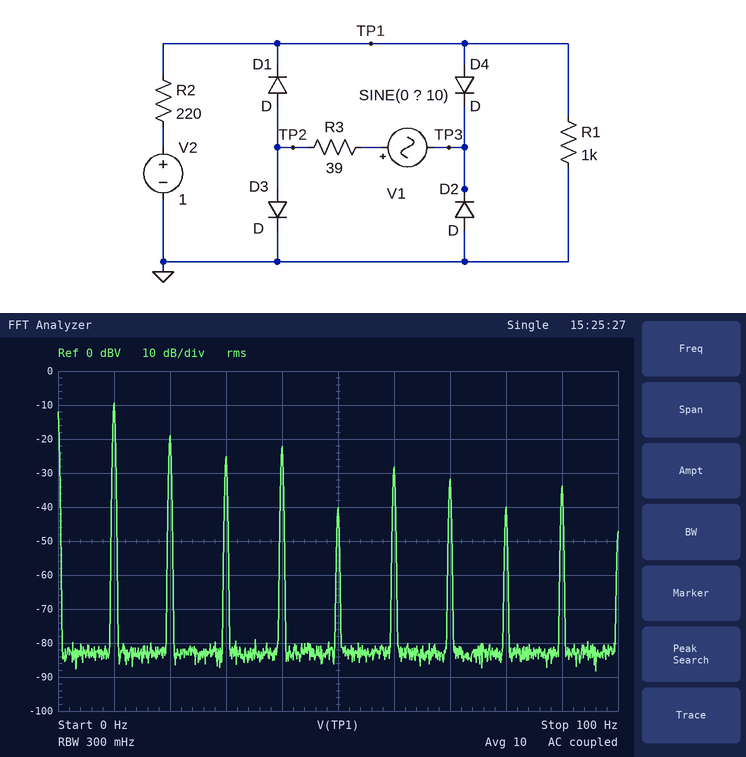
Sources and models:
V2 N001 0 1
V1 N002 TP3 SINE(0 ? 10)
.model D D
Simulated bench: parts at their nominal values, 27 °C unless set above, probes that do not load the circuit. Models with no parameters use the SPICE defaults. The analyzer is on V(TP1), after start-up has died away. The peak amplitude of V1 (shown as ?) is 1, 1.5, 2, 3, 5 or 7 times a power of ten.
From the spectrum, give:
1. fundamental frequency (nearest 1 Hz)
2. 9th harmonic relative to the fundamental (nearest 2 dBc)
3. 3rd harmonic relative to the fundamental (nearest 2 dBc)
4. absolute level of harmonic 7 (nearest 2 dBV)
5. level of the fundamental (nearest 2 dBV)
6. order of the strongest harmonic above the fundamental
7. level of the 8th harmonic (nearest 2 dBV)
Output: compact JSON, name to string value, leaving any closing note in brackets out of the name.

{"fundamental frequency": "10 Hz", "9th harmonic relative to the fundamental": "-24 dBc", "3rd harmonic relative to the fundamental": "-16 dBc", "absolute level of harmonic 7": "-32 dBV", "level of the fundamental": "-10 dBV", "order of the strongest harmonic above the fundamental": "2", "level of the 8th harmonic": "-40 dBV"}
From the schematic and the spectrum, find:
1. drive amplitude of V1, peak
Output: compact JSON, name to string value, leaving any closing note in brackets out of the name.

{"drive amplitude of V1, peak": "3 V"}
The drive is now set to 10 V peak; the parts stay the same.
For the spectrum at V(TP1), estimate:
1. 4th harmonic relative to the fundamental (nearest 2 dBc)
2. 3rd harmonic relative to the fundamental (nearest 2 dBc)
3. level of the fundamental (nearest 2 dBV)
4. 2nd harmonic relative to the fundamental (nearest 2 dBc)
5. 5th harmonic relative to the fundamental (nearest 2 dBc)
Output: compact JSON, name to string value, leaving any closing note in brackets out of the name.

{"4th harmonic relative to the fundamental": "-20 dBc", "3rd harmonic relative to the fundamental": "-10 dBc", "level of the fundamental": "-8 dBV", "2nd harmonic relative to the fundamental": "-20 dBc", "5th harmonic relative to the fundamental": "-16 dBc"}
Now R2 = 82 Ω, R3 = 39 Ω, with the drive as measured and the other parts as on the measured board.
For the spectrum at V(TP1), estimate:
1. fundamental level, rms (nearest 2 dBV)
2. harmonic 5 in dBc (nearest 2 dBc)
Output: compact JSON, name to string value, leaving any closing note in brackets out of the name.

{"fundamental level, rms": "-8 dBV", "harmonic 5 in dBc": "-24 dBc"}
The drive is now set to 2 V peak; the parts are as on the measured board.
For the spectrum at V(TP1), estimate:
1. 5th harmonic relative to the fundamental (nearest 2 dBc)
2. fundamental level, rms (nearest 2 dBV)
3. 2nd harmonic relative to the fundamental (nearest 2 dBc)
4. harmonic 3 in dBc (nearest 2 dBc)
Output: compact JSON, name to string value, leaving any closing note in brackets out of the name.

{"5th harmonic relative to the fundamental": "-18 dBc", "fundamental level, rms": "-10 dBV", "2nd harmonic relative to the fundamental": "-6 dBc", "harmonic 3 in dBc": "-36 dBc"}
